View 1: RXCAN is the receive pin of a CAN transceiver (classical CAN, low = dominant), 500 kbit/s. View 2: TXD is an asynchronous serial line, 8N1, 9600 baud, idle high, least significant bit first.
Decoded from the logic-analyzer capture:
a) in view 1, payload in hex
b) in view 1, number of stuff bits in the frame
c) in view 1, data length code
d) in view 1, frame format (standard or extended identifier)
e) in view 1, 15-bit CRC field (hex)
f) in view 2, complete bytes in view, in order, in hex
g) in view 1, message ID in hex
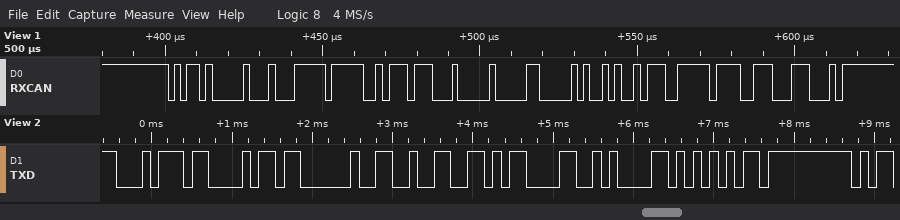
FF D7 71 00 20 4A 5C FF
7
8
standard
0x4E38
0x74 0x68 0x20 0x32 0x0D 0x0A 0x55 0xFF
0x5A0
